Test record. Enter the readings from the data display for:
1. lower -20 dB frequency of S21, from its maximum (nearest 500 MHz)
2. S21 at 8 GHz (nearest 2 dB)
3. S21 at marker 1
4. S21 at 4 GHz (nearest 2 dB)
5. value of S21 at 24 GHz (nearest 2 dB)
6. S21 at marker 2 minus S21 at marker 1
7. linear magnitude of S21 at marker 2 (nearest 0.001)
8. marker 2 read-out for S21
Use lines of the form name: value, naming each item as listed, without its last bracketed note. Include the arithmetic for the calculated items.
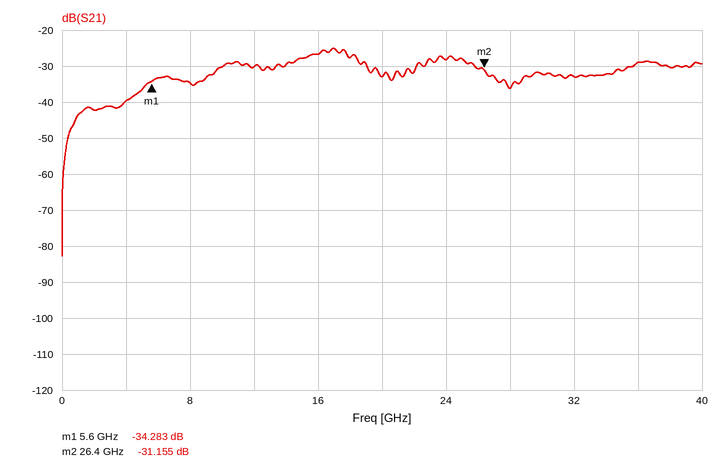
lower -20 dB frequency of S21, from its maximum: 1.0 GHz
S21 at 8 GHz: -34 dB
S21 at marker 1: -34.283 dB
S21 at 4 GHz: -40 dB
value of S21 at 24 GHz: -28 dB
S21 at marker 2 minus S21 at marker 1: -31.155 − (-34.283) = 3.128 dB
linear magnitude of S21 at marker 2: 10^(-31.155/20) ≈ 0.028
marker 2 read-out for S21: -31.155 dB
